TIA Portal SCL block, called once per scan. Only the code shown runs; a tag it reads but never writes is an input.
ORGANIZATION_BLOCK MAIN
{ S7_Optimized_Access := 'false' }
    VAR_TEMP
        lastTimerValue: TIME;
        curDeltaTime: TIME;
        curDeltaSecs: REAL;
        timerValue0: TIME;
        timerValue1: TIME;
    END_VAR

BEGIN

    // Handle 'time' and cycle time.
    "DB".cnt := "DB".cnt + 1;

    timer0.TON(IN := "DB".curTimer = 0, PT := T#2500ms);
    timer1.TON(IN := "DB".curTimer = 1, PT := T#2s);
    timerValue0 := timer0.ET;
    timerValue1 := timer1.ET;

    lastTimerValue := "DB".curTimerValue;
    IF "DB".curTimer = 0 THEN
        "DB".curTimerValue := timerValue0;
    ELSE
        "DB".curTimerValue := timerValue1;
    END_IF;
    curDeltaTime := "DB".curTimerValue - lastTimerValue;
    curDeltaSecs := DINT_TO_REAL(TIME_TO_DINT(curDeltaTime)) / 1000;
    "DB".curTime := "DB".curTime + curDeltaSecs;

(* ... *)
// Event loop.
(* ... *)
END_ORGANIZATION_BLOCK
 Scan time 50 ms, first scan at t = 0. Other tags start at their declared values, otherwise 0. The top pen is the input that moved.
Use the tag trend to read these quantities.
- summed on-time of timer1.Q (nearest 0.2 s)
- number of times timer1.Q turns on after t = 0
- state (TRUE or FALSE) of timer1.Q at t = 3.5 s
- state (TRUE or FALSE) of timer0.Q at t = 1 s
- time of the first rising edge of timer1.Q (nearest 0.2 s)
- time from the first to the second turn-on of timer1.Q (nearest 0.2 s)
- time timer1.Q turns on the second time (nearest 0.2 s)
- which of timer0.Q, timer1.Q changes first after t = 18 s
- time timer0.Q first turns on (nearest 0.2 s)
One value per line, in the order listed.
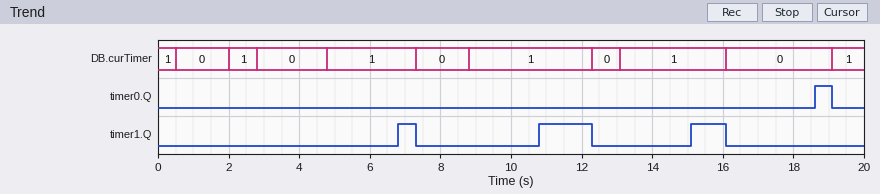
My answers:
3.0 s
3
FALSE
FALSE
6.8 s
4.0 s
10.8 s
timer0.Q
18.6 s
